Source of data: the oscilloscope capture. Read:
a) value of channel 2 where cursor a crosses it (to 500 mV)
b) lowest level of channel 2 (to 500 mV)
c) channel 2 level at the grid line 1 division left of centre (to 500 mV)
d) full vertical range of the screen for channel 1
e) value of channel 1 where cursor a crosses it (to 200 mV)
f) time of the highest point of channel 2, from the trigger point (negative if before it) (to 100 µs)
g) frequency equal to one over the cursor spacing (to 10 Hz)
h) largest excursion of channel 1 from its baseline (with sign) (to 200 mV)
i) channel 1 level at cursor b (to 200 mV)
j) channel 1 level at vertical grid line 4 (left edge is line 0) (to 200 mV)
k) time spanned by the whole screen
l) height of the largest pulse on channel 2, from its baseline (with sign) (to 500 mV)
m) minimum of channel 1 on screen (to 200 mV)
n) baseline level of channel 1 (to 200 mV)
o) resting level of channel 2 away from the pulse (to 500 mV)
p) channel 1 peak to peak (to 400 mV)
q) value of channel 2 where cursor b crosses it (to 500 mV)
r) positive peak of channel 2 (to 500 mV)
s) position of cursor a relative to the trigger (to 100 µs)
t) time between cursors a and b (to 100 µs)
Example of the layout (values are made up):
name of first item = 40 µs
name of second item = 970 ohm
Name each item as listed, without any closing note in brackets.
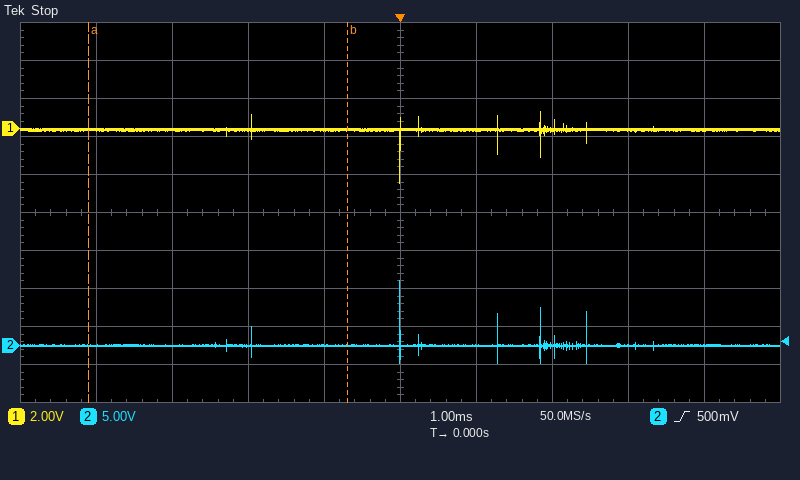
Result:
value of channel 2 where cursor a crosses it = 0.0 V
lowest level of channel 2 = -2.0 V
channel 2 level at the grid line 1 division left of centre = 0.0 V
full vertical range of the screen for channel 1 = 20 V
value of channel 1 where cursor a crosses it = 0.0 V
time of the highest point of channel 2, from the trigger point (negative if before it) = 0.0 ms
frequency equal to one over the cursor spacing = 290 Hz
largest excursion of channel 1 from its baseline (with sign) = -2.8 V
channel 1 level at cursor b = 0.0 V
channel 1 level at vertical grid line 4 (left edge is line 0) = 0.0 V
time spanned by the whole screen = 10 ms
height of the largest pulse on channel 2, from its baseline (with sign) = +8.5 V
minimum of channel 1 on screen = -2.8 V
baseline level of channel 1 = 0.0 V
resting level of channel 2 away from the pulse = 0.0 V
channel 1 peak to peak = 3.6 V
value of channel 2 where cursor b crosses it = 0.0 V
positive peak of channel 2 = 8.5 V
position of cursor a relative to the trigger = -4.1 ms
time between cursors a and b = 3.4 ms
